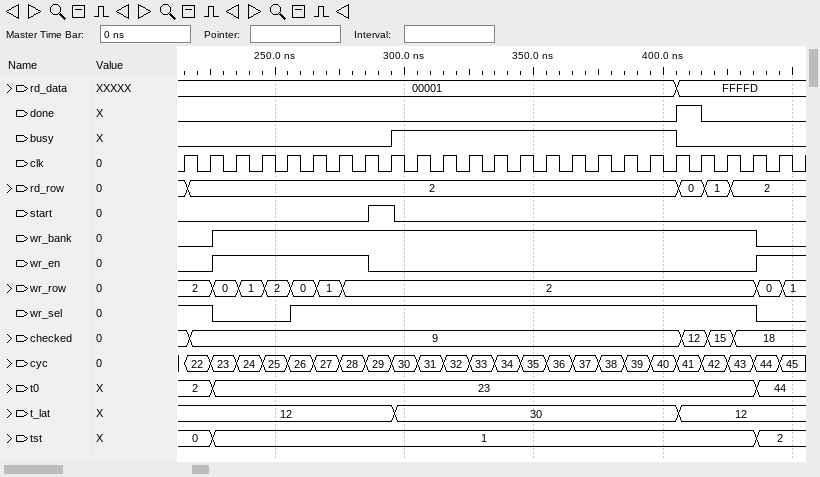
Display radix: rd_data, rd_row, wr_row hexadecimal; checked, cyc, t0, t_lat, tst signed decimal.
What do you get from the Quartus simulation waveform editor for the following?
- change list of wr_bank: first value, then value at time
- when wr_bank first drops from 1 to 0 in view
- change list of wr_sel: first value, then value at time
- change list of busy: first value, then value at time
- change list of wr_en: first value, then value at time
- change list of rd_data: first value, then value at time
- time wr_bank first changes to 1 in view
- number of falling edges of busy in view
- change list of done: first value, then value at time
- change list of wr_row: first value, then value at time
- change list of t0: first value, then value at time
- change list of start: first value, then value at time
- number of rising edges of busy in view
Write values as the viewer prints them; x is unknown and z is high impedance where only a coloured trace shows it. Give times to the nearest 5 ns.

0, 1 at 225 ns, 0 at 435 ns
435 ns
1, 0 at 225 ns, 1 at 255 ns, 0 at 435 ns
0, 1 at 295 ns, 0 at 405 ns
0, 1 at 225 ns, 0 at 285 ns, 1 at 435 ns
00001, FFFFD at 405 ns
225 ns
1
0, 1 at 405 ns, 0 at 415 ns
2, 0 at 225 ns, 1 at 235 ns, 2 at 245 ns, 0 at 255 ns, 1 at 265 ns, 2 at 275 ns, 0 at 435 ns, 1 at 445 ns
2, 23 at 225 ns, 44 at 435 ns
0, 1 at 285 ns, 0 at 295 ns
1
